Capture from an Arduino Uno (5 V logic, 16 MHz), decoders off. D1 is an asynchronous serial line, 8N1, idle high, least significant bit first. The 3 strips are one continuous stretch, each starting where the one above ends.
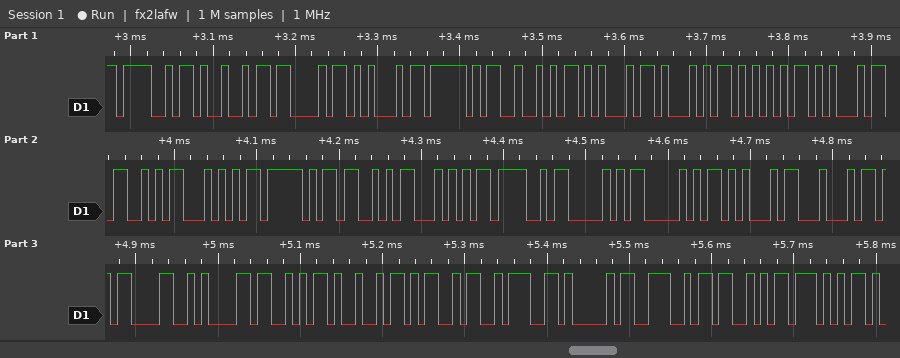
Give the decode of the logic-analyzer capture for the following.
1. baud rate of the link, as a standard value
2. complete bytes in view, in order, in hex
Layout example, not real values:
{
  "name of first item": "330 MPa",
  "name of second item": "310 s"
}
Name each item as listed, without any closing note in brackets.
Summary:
{
  "baud rate of the link, as a standard value": "115200 baud",
  "complete bytes in view, in order, in hex": "4F 49 43 45 5F 52 45 51 55 45 53 54 5F 53 54 4F 50 50 45 44 0D 0A 53 49 4D 3A 41 4E 53 57"
}
